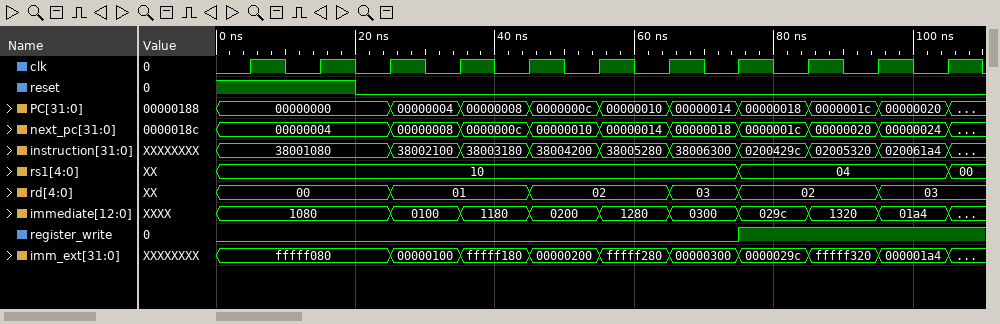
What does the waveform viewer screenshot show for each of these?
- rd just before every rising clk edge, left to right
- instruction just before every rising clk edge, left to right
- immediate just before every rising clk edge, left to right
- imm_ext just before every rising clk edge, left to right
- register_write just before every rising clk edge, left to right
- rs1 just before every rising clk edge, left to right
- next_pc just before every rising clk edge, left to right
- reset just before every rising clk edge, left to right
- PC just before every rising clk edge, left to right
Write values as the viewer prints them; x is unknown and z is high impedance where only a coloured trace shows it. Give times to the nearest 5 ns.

00, 00, 00, 01, 01, 02, 02, 03, 02, 02, 03
38001080, 38001080, 38001080, 38002100, 38003180, 38004200, 38005280, 38006300, 0200429c, 02005320, 020061a4
1080, 1080, 1080, 0100, 1180, 0200, 1280, 0300, 029c, 1320, 01a4
fffff080, fffff080, fffff080, 00000100, fffff180, 00000200, fffff280, 00000300, 0000029c, fffff320, 000001a4
0 0 0 0 0 0 0 0 1 1 1
10, 10, 10, 10, 10, 10, 10, 10, 04, 04, 04
00000004, 00000004, 00000004, 00000008, 0000000c, 00000010, 00000014, 00000018, 0000001c, 00000020, 00000024
1 1 0 0 0 0 0 0 0 0 0
00000000, 00000000, 00000000, 00000004, 00000008, 0000000c, 00000010, 00000014, 00000018, 0000001c, 00000020
